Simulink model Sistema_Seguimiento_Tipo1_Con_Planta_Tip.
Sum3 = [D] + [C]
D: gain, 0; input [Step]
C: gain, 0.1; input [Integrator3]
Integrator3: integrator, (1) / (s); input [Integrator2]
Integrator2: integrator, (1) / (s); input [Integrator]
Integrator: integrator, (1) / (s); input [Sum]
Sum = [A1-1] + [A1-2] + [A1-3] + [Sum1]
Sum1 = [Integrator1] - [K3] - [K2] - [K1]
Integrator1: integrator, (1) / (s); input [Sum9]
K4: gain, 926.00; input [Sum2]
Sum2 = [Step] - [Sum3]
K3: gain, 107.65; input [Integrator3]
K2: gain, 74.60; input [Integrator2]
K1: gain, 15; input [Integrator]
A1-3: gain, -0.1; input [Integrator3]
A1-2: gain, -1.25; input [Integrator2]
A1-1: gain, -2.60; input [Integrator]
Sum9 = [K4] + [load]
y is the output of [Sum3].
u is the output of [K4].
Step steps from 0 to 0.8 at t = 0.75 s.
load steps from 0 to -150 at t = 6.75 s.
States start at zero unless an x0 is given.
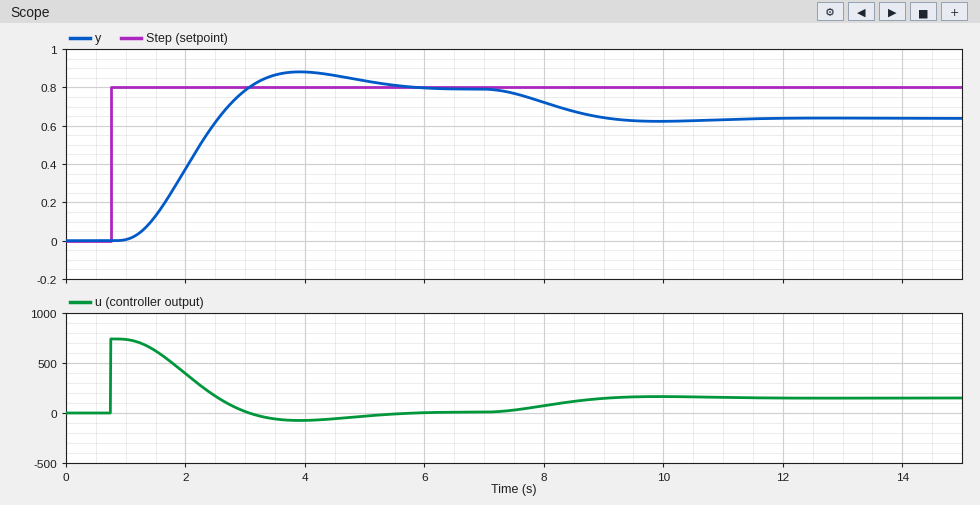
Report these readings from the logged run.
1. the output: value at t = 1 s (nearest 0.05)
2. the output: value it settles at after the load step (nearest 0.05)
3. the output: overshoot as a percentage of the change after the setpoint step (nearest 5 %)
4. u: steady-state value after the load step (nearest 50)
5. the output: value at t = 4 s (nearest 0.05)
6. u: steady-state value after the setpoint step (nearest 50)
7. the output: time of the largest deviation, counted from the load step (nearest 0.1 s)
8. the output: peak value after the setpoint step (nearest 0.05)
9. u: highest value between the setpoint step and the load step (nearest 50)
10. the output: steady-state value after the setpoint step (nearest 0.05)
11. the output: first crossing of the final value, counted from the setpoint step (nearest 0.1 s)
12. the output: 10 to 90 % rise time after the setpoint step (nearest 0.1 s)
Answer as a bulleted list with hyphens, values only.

- 0.00
- 0.65
- 10 %
- 150
- 0.90
- 0
- 3.2 s
- 0.90
- 750
- 0.80
- 2.3 s
- 1.4 s
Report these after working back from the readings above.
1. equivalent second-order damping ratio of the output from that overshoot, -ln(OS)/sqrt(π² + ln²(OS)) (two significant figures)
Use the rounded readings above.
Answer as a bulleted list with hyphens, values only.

- 0.59
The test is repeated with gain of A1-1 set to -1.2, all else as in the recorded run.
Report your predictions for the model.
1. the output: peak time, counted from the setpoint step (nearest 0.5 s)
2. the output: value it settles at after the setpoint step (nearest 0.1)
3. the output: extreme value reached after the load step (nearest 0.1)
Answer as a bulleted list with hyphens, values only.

- 3.0 s
- 0.8
- 0.6
